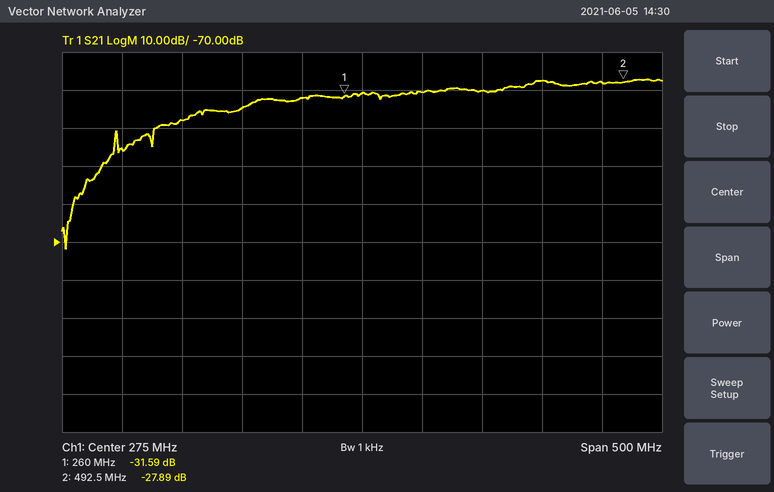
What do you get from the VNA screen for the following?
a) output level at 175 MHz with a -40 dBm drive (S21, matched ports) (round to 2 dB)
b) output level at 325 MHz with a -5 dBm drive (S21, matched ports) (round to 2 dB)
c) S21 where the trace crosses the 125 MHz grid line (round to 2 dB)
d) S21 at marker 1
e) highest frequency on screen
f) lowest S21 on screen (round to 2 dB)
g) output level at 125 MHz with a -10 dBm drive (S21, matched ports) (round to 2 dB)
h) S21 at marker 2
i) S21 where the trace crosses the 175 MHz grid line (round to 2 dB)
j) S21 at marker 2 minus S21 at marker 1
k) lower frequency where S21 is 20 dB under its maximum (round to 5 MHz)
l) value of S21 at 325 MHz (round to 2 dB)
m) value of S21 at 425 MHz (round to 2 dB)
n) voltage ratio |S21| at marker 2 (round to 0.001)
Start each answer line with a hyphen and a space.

- -74 dBm
- -36 dBm
- -38 dB
- -31.59 dB
- 525 MHz
- -72 dB
- -48 dBm
- -27.89 dB
- -34 dB
- 3.70 dB
- 65 MHz
- -30 dB
- -28 dB
- 0.040
